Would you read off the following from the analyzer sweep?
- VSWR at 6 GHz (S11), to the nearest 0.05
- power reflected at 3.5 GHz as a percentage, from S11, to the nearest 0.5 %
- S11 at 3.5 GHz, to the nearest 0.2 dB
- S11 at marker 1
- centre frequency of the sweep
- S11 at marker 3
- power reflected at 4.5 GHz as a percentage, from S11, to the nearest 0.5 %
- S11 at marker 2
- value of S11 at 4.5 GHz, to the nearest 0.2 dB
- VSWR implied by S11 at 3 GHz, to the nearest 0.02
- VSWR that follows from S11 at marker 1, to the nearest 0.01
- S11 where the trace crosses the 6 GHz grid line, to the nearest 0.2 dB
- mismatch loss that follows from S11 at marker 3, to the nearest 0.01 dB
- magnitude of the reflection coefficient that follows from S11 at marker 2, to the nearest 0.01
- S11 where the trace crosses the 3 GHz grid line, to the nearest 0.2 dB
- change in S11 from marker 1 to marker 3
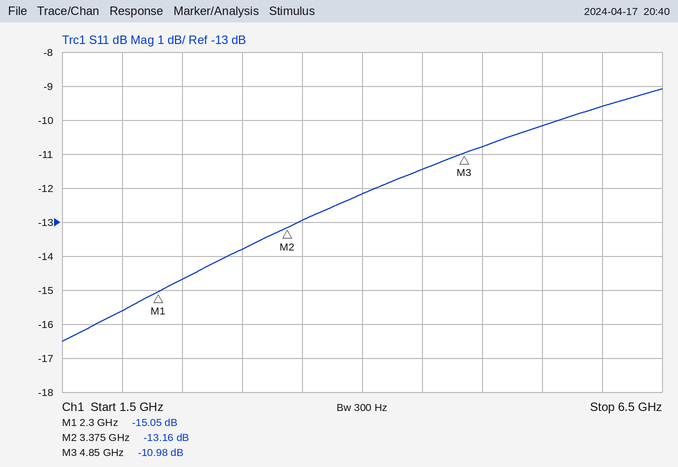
2.00
5.0 %
-13.0 dB
-15.05 dB
4 GHz
-10.98 dB
7.0 %
-13.16 dB
-11.4 dB
1.52
1.43
-9.6 dB
0.36 dB
0.22
-13.8 dB
4.07 dB
